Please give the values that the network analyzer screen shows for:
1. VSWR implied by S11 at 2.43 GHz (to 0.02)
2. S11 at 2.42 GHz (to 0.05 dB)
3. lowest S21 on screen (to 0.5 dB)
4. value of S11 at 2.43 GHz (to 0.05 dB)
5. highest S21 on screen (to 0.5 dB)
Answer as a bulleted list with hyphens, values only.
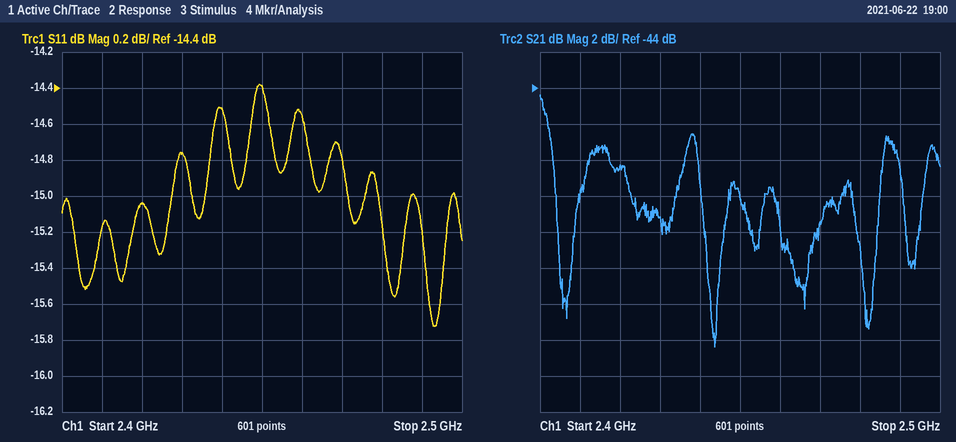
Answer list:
- 1.44
- -15.05 dB
- -58.5 dB
- -14.75 dB
- -44.5 dB
